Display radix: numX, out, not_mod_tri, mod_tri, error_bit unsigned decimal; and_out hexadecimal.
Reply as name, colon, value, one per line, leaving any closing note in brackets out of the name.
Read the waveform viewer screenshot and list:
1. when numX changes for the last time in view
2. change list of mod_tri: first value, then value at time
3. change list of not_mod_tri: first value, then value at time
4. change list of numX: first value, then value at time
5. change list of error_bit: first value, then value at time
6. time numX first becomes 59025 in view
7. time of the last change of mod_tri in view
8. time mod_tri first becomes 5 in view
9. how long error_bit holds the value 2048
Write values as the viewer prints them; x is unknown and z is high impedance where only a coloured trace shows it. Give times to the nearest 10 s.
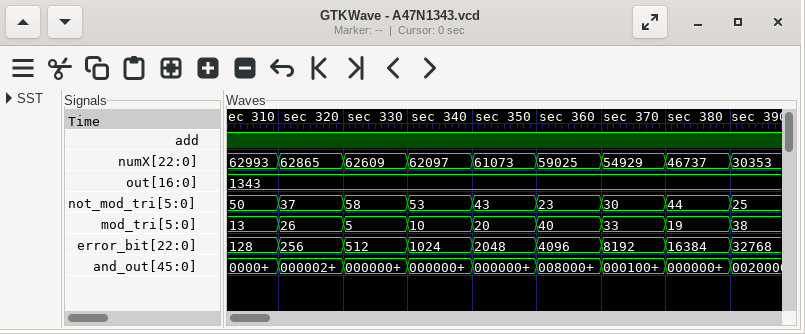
when numX changes for the last time in view: 380 s
change list of mod_tri: first value, then value at time: 13, 26 at 310 s, 5 at 320 s, 10 at 330 s, 20 at 340 s, 40 at 350 s, 33 at 360 s, 19 at 370 s, 38 at 380 s
change list of not_mod_tri: first value, then value at time: 50, 37 at 310 s, 58 at 320 s, 53 at 330 s, 43 at 340 s, 23 at 350 s, 30 at 360 s, 44 at 370 s, 25 at 380 s
change list of numX: first value, then value at time: 62993, 62865 at 310 s, 62609 at 320 s, 62097 at 330 s, 61073 at 340 s, 59025 at 350 s, 54929 at 360 s, 46737 at 370 s, 30353 at 380 s
change list of error_bit: first value, then value at time: 128, 256 at 310 s, 512 at 320 s, 1024 at 330 s, 2048 at 340 s, 4096 at 350 s, 8192 at 360 s, 16384 at 370 s, 32768 at 380 s
time numX first becomes 59025 in view: 350 s
time of the last change of mod_tri in view: 380 s
time mod_tri first becomes 5 in view: 320 s
how long error_bit holds the value 2048: 10 s
